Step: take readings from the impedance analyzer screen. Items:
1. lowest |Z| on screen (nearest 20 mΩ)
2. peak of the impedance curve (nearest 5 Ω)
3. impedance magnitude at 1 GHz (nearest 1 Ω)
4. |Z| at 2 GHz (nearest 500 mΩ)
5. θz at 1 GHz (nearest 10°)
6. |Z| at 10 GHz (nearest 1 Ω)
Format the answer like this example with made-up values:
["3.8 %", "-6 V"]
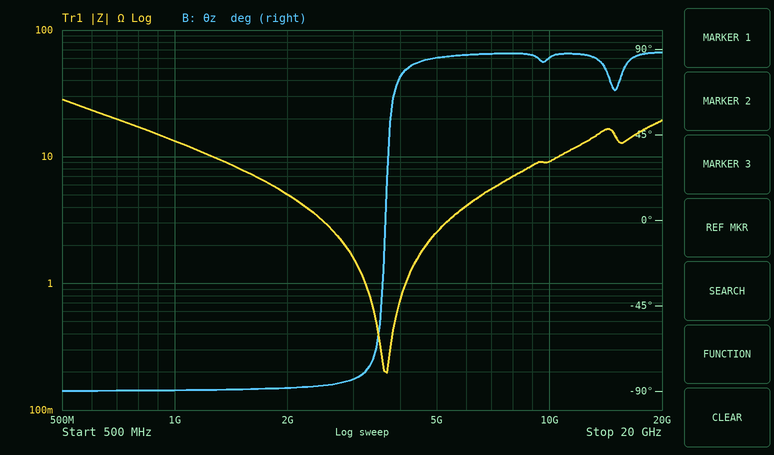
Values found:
["200 mΩ", "30 Ω", "13 Ω", "5.0 Ω", "-90°", "9 Ω"]
